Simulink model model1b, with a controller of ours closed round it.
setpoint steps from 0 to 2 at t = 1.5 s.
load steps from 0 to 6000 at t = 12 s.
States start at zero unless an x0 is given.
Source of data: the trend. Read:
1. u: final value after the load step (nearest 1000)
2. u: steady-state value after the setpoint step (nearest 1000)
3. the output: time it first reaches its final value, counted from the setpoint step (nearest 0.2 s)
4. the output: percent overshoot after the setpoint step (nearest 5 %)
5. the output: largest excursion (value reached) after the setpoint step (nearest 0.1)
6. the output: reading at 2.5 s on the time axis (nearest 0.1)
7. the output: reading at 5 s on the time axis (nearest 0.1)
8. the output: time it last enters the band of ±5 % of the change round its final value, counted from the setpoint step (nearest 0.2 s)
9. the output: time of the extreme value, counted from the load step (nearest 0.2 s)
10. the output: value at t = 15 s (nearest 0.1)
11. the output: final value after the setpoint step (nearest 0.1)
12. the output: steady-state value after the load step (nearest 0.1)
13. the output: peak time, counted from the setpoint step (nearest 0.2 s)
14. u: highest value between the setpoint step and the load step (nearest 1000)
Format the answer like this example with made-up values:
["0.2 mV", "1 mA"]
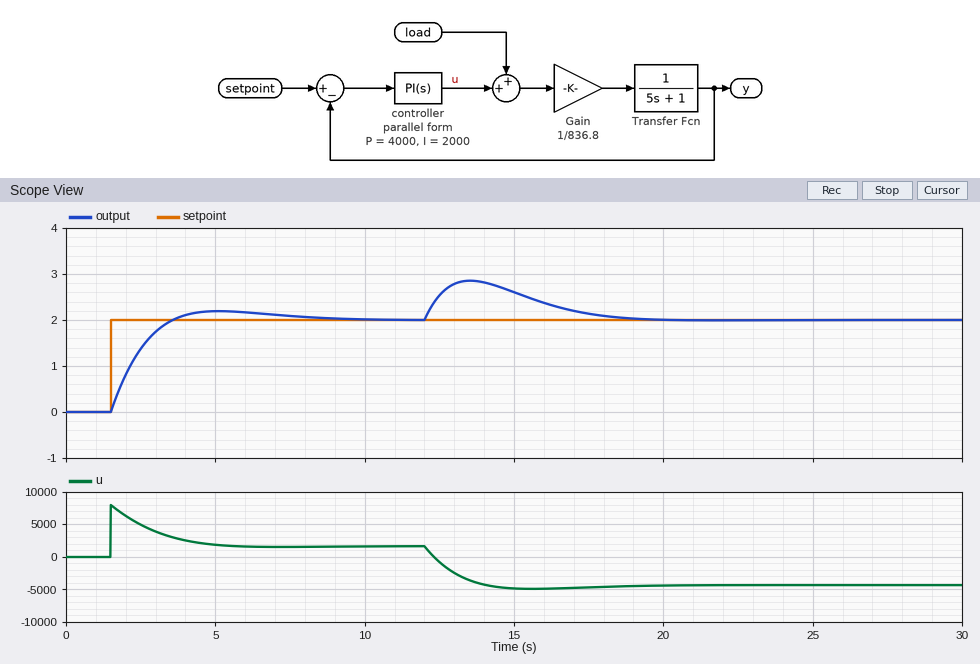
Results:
["-4000", "2000", "2.0 s", "10 %", "2.2", "1.4", "2.2", "5.8 s", "1.6 s", "2.6", "2.0", "2.0", "3.6 s", "8000"]
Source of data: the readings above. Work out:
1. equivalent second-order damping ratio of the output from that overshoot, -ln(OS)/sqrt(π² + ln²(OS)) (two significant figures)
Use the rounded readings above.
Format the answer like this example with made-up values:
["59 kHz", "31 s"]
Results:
["0.59"]
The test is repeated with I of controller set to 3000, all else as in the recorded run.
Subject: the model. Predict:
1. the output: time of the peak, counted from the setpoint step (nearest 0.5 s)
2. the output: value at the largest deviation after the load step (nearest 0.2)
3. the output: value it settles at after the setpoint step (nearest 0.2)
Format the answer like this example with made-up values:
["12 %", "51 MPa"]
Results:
["3.0 s", "2.8", "2.0"]
